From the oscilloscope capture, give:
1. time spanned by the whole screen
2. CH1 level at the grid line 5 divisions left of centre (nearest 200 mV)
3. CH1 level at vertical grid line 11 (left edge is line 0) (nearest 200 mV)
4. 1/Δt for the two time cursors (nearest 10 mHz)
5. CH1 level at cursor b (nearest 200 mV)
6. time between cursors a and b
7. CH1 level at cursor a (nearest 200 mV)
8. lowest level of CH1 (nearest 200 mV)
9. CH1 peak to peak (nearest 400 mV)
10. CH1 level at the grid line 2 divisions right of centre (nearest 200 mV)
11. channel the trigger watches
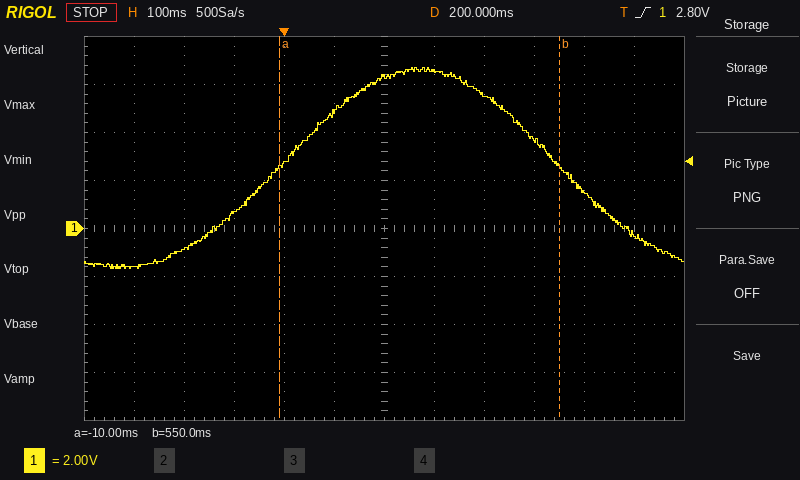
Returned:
1.2 s
-1.6 V
-200 mV
1.79 Hz
2.6 V
560 ms
2.6 V
-1.6 V
8.4 V
5.6 V
CH1
